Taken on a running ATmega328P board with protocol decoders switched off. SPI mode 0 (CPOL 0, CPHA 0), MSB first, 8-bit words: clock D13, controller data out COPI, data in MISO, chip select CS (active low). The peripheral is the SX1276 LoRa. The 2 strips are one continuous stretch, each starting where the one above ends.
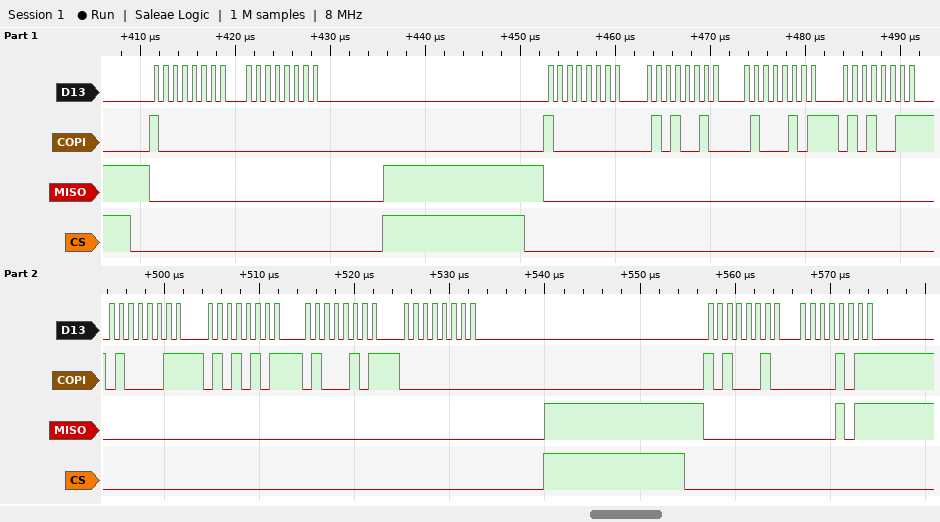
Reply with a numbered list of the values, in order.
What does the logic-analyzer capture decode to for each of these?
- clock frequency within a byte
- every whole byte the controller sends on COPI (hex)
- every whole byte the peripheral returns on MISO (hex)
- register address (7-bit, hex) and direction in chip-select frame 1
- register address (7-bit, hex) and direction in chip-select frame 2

1. 1 MHz
2. 80 00 80 52 45 53 43 55 45 00 A2 0B
3. 00 00 00 00 00 00 00 00 00 00 00 0B
4. 0x00 write
5. 0x00 write
